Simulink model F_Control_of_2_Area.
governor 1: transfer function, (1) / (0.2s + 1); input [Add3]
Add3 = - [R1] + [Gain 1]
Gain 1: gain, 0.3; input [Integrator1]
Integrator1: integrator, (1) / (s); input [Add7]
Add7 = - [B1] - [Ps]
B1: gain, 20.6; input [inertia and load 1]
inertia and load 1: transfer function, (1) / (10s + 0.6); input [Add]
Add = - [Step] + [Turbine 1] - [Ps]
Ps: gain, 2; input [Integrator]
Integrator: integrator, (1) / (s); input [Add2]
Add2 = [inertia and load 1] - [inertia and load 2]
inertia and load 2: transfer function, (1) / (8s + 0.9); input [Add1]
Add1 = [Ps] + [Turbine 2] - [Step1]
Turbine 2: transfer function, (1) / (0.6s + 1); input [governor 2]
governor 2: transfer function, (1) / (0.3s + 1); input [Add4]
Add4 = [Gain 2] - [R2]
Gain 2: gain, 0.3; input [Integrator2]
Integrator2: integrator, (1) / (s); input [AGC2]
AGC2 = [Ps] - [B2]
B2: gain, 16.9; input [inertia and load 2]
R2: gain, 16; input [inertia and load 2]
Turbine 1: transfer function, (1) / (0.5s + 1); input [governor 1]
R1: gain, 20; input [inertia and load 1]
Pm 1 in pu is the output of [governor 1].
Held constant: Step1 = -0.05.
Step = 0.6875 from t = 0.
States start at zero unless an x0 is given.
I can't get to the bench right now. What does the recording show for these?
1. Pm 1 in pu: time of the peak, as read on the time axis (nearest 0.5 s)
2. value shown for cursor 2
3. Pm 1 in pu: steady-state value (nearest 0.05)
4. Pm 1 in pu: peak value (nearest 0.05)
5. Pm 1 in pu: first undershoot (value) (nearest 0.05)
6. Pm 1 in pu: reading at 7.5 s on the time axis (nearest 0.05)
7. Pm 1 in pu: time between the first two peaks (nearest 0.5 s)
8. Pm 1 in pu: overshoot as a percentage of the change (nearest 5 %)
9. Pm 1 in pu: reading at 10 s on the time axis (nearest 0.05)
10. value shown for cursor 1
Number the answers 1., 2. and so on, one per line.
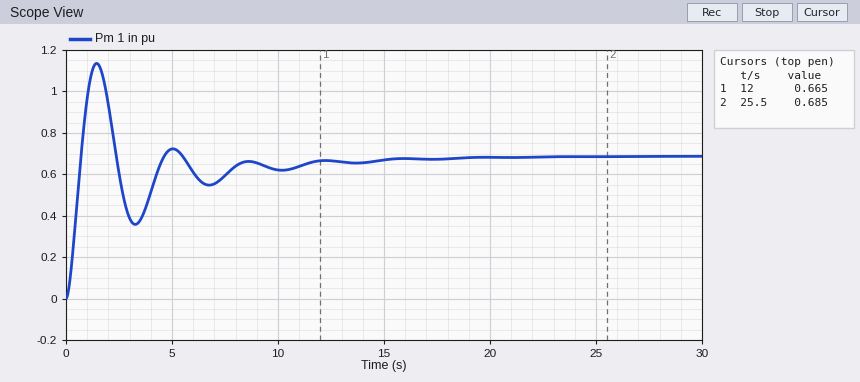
1. 1.5 s
2. 0.685
3. 0.70
4. 1.15
5. 0.35
6. 0.60
7. 3.5 s
8. 65 %
9. 0.60
10. 0.665
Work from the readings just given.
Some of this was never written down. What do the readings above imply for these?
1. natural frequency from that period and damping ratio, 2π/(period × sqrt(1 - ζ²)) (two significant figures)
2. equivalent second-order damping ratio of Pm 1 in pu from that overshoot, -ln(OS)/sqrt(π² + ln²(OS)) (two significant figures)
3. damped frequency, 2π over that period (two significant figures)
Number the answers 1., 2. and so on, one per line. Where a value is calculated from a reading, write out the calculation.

1. 2π / (3.5 × sqrt(1 - 0.14²)) = 1.8 rad/s
2. ln(0.65) = -0.431; 0.431 / sqrt(9.870 + 0.186) = 0.14
3. 2π / 3.5 = 1.8 rad/s
